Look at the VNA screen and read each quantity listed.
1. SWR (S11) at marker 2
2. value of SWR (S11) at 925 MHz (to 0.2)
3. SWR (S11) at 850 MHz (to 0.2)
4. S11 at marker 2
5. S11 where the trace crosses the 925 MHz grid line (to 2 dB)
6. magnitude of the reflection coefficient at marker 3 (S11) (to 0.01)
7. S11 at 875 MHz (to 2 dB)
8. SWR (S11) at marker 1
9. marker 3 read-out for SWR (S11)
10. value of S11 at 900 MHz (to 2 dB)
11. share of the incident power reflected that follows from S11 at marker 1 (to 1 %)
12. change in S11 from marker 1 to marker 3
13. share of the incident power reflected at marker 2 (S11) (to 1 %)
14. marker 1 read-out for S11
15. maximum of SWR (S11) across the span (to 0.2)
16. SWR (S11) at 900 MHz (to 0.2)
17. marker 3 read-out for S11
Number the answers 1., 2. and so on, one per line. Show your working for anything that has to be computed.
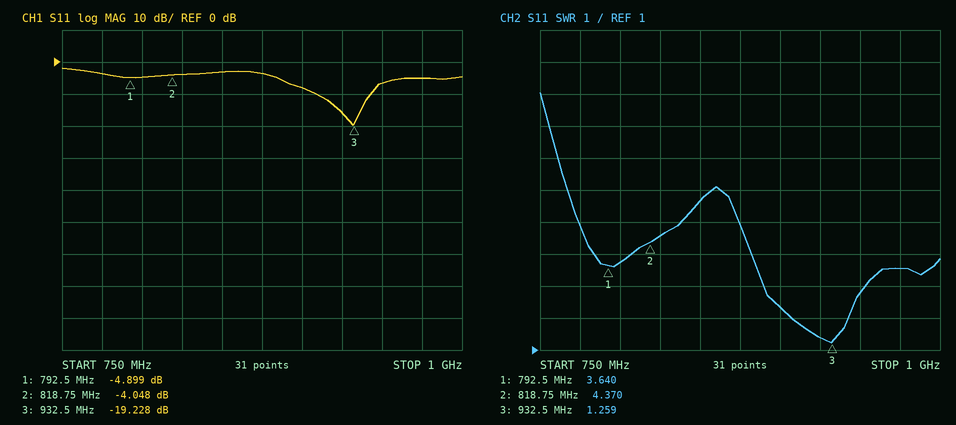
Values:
1. 4.370
2. 1.4
3. 5.6
4. -4.048 dB
5. -16 dB
6. 10^(-19.228/20) ≈ 0.11
7. -4 dB
8. 3.640
9. 1.259
10. -8 dB
11. 10^(-4.899/10) ≈ 32 %
12. -19.228 − (-4.899) = -14.329 dB
13. 10^(-4.048/10) ≈ 39 %
14. -4.899 dB
15. 9.0
16. 2.4
17. -19.228 dB
